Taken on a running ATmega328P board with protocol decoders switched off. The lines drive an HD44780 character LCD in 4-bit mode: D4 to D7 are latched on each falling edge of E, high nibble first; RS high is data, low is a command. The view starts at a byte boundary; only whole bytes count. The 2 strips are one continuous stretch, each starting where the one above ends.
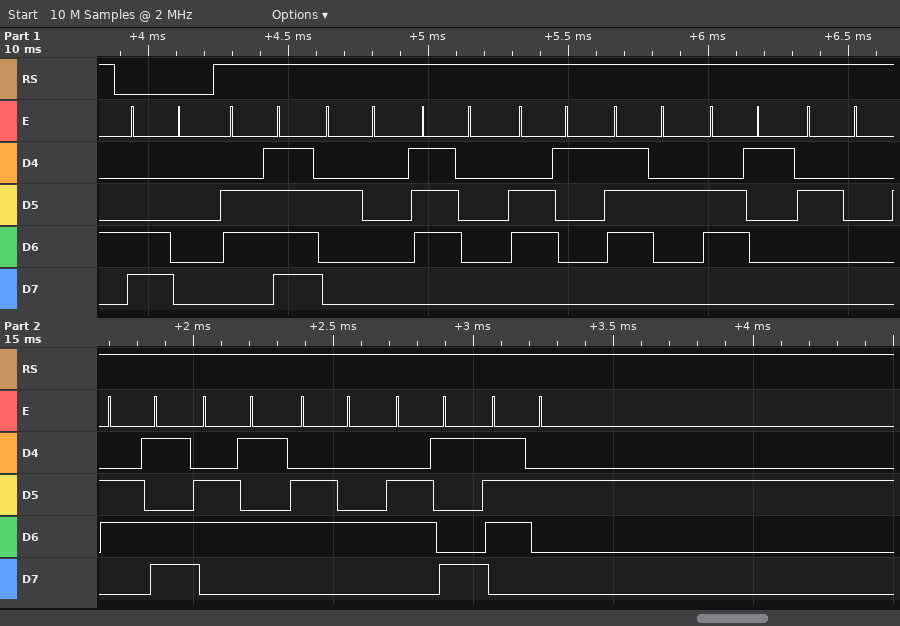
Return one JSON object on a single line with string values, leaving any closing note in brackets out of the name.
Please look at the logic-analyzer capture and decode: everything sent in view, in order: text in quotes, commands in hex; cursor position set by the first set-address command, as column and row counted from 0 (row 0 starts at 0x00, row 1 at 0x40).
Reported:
{"everything sent in view, in order: text in quotes, commands in hex": "0xC0 \"o para medir\"", "cursor position set by the first set-address command, as column and row counted from 0": "column 0, row 1"}
